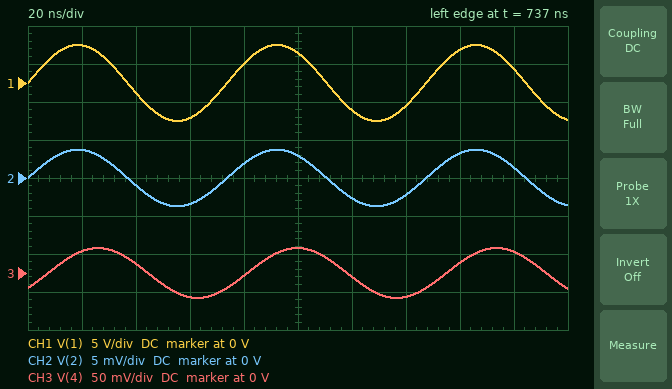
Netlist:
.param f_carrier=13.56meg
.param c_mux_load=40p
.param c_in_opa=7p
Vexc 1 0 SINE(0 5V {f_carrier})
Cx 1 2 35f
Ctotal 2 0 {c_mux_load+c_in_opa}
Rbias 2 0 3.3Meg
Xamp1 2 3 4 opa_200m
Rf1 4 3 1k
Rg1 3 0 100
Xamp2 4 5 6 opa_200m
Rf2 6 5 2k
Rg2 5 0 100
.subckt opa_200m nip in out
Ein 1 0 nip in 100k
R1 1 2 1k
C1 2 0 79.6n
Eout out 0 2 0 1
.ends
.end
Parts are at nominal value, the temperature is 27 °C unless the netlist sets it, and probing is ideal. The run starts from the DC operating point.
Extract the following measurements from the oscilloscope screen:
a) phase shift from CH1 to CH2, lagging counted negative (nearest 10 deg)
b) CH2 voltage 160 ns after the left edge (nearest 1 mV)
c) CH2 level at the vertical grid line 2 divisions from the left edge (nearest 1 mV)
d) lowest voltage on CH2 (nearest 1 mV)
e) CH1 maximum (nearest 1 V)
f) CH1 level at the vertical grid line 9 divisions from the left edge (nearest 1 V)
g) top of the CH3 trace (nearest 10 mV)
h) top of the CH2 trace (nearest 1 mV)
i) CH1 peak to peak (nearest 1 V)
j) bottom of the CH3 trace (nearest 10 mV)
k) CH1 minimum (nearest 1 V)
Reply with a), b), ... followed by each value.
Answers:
a) 0 deg
b) 3 mV
c) -1 mV
d) -4 mV
e) 5 V
f) 2 V
g) 30 mV
h) 4 mV
i) 10 V
j) -30 mV
k) -5 V
